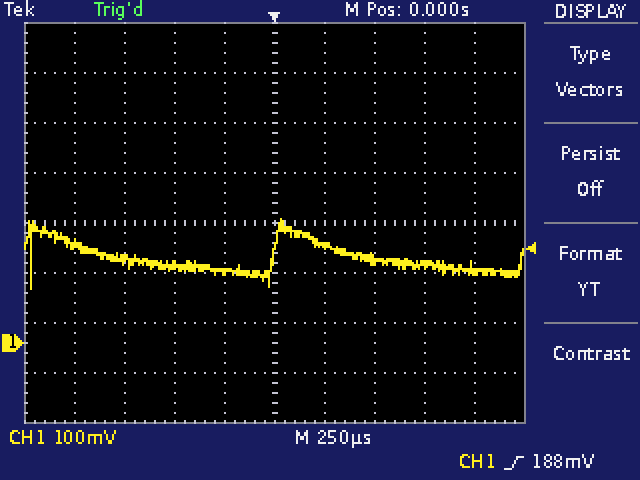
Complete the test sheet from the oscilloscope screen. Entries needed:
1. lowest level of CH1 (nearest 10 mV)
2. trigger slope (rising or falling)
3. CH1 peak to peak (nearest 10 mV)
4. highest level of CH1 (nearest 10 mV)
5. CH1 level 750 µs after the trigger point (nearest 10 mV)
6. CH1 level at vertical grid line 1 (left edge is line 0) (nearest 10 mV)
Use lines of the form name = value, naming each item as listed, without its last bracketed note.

lowest level of CH1 = 110 mV
trigger slope = rising
CH1 peak to peak = 140 mV
highest level of CH1 = 250 mV
CH1 level 750 µs after the trigger point = 160 mV
CH1 level at vertical grid line 1 (left edge is line 0) = 200 mV
